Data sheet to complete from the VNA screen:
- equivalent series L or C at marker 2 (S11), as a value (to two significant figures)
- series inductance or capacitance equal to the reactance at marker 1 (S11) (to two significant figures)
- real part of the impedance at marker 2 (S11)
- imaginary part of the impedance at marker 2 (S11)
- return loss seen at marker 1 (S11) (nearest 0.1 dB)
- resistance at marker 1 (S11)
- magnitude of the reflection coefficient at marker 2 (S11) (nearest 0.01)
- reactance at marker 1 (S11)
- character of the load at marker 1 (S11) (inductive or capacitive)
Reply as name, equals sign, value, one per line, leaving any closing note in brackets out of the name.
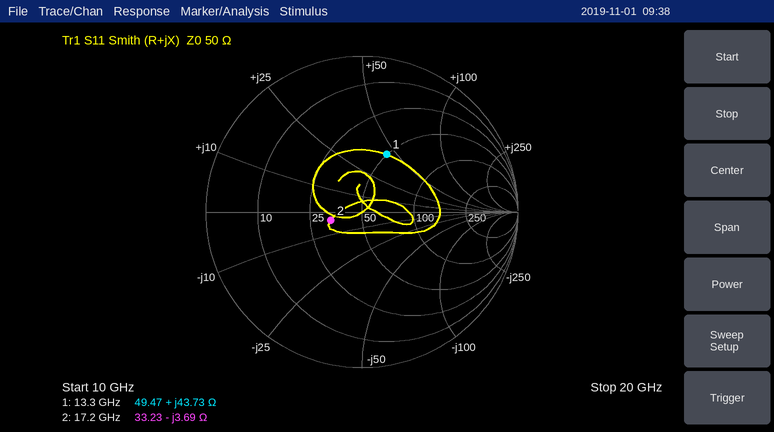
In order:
equivalent series L or C at marker 2 (S11), as a value = 2.5 pF
series inductance or capacitance equal to the reactance at marker 1 (S11) = 520 pH
real part of the impedance at marker 2 = 33.23 Ω
imaginary part of the impedance at marker 2 = -3.69 Ω
return loss seen at marker 1 (S11) = 7.9 dB
resistance at marker 1 = 49.47 Ω
magnitude of the reflection coefficient at marker 2 (S11) = 0.21
reactance at marker 1 = +43.73 Ω
character of the load at marker 1 (S11) = inductive
